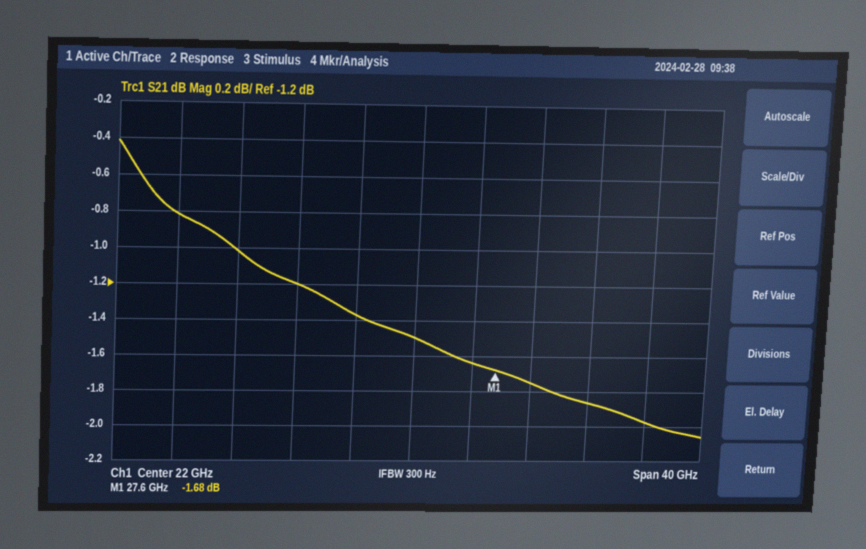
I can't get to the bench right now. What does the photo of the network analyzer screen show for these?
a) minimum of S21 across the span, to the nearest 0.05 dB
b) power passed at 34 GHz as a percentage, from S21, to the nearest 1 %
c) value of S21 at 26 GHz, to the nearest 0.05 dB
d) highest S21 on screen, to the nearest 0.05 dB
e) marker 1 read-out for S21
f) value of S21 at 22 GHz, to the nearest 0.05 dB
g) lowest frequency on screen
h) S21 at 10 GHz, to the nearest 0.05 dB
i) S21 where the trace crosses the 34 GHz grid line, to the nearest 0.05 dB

-2.05 dB
65 %
-1.65 dB
-0.40 dB
-1.68 dB
-1.50 dB
2 GHz
-1.00 dB
-1.85 dB
